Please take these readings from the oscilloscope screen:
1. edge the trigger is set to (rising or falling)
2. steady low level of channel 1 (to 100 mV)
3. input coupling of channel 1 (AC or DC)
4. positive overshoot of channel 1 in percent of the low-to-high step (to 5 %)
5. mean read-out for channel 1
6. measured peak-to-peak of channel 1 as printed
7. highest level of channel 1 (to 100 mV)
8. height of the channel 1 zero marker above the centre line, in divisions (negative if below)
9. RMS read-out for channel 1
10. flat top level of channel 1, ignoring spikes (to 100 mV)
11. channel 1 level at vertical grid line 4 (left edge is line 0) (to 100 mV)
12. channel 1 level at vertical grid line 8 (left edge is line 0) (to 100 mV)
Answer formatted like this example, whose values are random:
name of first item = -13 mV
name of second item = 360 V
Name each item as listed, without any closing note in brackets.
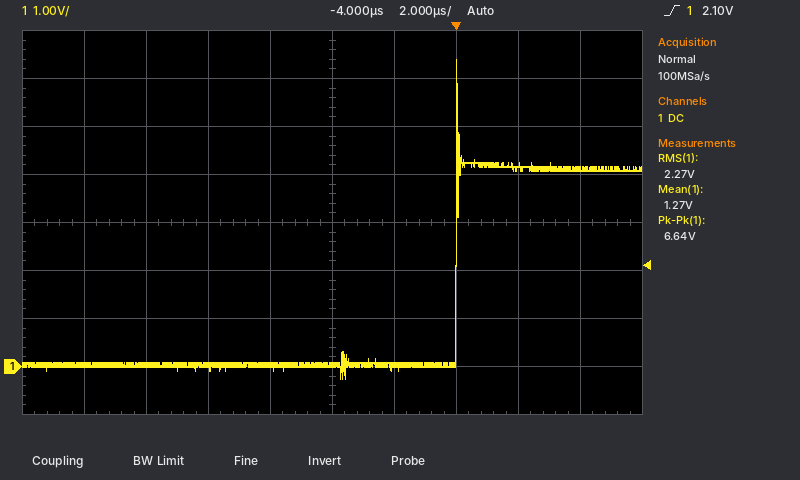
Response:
edge the trigger is set to = rising
steady low level of channel 1 = 0.0 V
input coupling of channel 1 = DC
positive overshoot of channel 1 in percent of the low-to-high step = 55 %
mean read-out for channel 1 = 1.27 V
measured peak-to-peak of channel 1 as printed = 6.64 V
highest level of channel 1 = 6.4 V
height of the channel 1 zero marker above the centre line, in divisions = -3.0 div
RMS read-out for channel 1 = 2.27 V
flat top level of channel 1, ignoring spikes = 4.1 V
channel 1 level at vertical grid line 4 (left edge is line 0) = 0.0 V
channel 1 level at vertical grid line 8 (left edge is line 0) = 4.2 V
